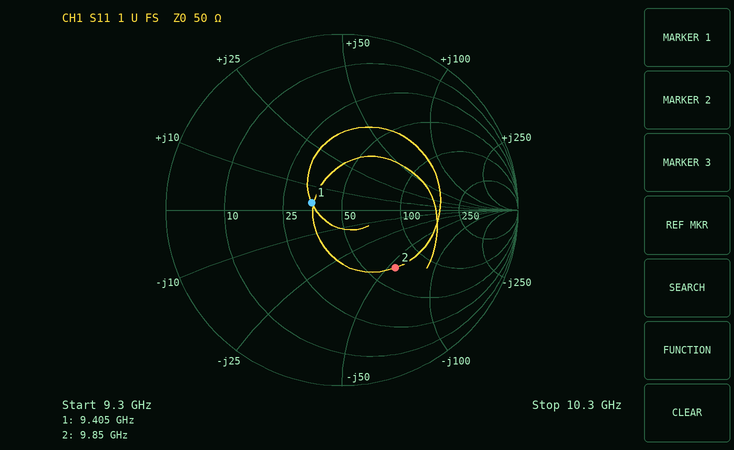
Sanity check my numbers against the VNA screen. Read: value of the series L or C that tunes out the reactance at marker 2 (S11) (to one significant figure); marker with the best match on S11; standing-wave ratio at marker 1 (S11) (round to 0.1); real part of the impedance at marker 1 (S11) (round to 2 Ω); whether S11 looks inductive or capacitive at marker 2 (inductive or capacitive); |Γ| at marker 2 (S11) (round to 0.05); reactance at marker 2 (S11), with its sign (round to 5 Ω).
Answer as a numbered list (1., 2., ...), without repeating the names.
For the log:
1. 900 pH
2. marker 1
3. 1.4
4. 36 Ω
5. capacitive
6. 0.45
7. -55 Ω
